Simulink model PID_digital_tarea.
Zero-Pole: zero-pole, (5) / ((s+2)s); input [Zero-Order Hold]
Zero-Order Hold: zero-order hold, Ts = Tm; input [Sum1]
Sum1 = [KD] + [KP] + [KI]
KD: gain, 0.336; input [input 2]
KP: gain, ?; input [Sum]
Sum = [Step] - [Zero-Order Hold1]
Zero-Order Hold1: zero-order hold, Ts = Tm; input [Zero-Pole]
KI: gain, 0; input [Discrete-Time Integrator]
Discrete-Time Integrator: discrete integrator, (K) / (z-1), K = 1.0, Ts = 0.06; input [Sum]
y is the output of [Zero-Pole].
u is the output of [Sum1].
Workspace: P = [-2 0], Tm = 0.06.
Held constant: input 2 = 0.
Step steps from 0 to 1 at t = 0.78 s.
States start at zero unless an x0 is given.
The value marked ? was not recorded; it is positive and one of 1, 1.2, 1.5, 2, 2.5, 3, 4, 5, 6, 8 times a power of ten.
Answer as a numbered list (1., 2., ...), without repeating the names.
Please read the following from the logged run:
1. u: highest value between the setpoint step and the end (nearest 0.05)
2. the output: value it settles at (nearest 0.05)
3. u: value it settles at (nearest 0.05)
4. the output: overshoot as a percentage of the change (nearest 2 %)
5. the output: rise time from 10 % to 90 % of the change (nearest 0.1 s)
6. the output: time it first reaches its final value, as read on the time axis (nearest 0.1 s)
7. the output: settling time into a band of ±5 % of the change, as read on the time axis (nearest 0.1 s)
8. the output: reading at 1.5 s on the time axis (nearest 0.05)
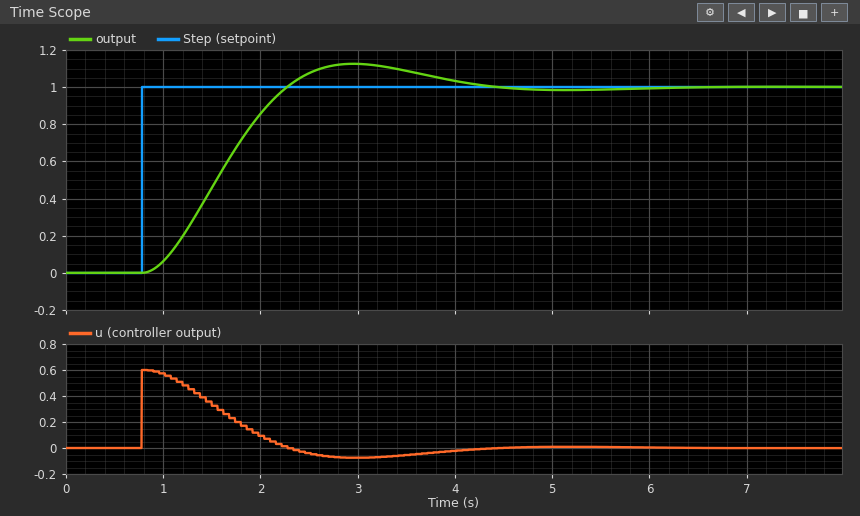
1. 0.60
2. 1.00
3. 0.00
4. 12 %
5. 1.0 s
6. 2.3 s
7. 3.8 s
8. 0.45
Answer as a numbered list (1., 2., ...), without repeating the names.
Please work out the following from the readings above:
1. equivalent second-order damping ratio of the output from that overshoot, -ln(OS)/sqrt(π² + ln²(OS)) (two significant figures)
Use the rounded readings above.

1. 0.56
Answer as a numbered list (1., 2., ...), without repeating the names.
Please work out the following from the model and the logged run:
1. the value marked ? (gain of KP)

1. 0.6
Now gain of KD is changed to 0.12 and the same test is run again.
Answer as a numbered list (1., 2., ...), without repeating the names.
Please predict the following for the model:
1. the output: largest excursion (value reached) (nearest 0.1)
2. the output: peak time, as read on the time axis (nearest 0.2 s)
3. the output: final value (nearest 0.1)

1. 1.1
2. 3.0 s
3. 1.0
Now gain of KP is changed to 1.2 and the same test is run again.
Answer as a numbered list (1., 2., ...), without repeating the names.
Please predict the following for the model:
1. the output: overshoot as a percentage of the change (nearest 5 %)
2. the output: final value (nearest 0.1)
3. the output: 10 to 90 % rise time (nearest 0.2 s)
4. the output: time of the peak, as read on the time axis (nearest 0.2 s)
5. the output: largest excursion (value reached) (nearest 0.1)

1. 30 %
2. 1.0
3. 0.6 s
4. 2.2 s
5. 1.3
